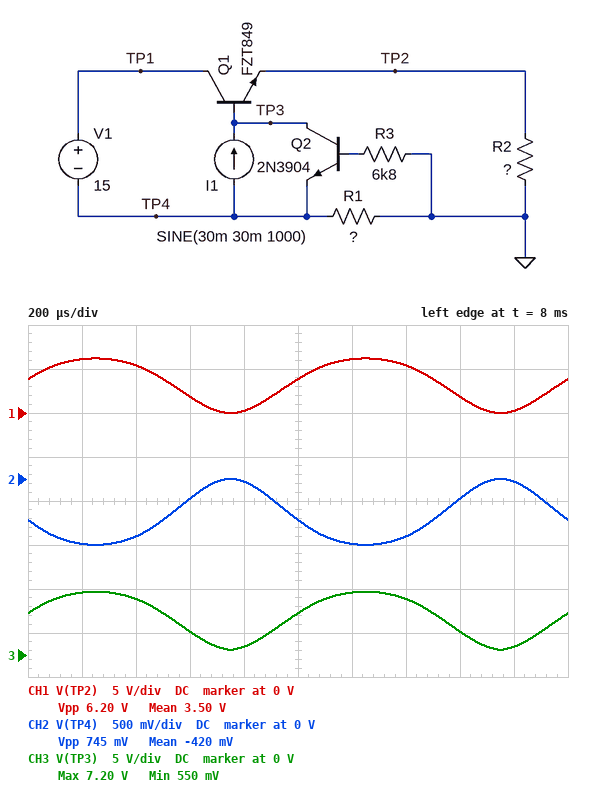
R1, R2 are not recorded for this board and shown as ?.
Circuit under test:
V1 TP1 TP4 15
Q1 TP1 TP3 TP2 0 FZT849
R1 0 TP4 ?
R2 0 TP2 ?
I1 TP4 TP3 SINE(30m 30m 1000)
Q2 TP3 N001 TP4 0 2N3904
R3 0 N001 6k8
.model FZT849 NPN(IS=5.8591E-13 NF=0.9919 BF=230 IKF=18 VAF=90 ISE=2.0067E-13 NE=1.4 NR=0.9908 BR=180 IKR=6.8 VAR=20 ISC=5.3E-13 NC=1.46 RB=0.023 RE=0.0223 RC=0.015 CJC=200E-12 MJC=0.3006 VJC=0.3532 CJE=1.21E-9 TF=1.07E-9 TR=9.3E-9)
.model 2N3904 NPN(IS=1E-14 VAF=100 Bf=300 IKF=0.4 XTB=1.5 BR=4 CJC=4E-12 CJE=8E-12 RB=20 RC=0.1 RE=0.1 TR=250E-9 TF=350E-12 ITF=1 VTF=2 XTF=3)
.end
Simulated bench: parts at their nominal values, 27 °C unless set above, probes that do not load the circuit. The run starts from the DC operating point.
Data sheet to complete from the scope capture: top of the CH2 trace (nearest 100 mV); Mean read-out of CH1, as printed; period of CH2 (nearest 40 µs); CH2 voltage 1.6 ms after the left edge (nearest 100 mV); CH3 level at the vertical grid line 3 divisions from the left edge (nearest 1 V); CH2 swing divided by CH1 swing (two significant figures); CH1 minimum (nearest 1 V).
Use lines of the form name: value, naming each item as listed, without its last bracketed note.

top of the CH2 trace: 0 V
Mean read-out of CH1, as printed: 3.50 V
period of CH2: 1.00 ms
CH2 voltage 1.6 ms after the left edge: -200 mV
CH3 level at the vertical grid line 3 divisions from the left edge: 3 V
CH2 swing divided by CH1 swing: 0.12
CH1 minimum: 0 V
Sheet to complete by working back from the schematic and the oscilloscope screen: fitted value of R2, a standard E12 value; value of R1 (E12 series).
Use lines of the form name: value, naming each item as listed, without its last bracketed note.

fitted value of R2, a standard E12 value: 0.68 Ω
value of R1: 0.082 Ω
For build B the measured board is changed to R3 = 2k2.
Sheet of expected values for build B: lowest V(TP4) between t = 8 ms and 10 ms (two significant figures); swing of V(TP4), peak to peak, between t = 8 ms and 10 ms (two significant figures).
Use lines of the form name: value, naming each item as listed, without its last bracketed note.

lowest V(TP4) between t = 8 ms and 10 ms: -730 mV
swing of V(TP4), peak to peak, between t = 8 ms and 10 ms: 730 mV
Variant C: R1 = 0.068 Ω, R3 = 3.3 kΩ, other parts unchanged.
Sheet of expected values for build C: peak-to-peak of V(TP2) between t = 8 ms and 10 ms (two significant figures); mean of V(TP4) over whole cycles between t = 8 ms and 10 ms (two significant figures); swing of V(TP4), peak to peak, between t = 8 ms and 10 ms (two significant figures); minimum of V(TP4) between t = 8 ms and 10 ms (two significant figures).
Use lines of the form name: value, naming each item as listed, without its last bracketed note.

peak-to-peak of V(TP2) between t = 8 ms and 10 ms: 6.4 V
mean of V(TP4) over whole cycles between t = 8 ms and 10 ms: -350 mV
swing of V(TP4), peak to peak, between t = 8 ms and 10 ms: 640 mV
minimum of V(TP4) between t = 8 ms and 10 ms: -640 mV
